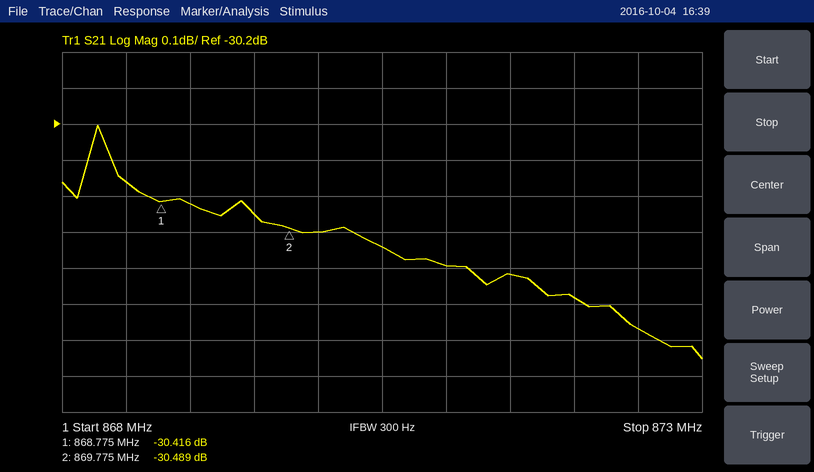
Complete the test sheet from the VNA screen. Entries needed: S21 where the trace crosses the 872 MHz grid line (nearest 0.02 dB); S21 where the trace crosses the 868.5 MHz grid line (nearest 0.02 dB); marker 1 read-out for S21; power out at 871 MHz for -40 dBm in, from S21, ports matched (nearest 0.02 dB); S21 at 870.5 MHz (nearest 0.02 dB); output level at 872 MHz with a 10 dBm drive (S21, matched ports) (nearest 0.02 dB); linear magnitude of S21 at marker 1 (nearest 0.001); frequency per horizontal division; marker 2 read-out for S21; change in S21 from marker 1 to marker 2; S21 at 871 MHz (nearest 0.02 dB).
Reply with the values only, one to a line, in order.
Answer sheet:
-30.68 dB
-30.36 dB
-30.416 dB
-70.60 dBm
-30.54 dB
-20.68 dBm
0.030
500 kHz
-30.489 dB
-0.073 dB
-30.60 dB
